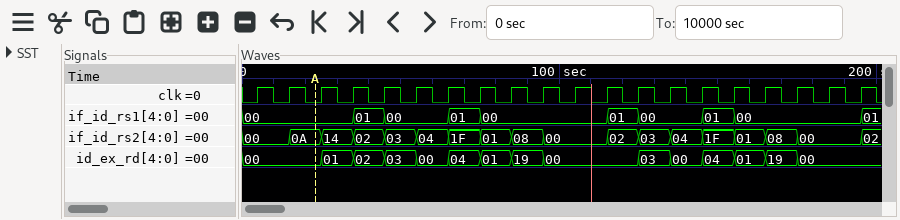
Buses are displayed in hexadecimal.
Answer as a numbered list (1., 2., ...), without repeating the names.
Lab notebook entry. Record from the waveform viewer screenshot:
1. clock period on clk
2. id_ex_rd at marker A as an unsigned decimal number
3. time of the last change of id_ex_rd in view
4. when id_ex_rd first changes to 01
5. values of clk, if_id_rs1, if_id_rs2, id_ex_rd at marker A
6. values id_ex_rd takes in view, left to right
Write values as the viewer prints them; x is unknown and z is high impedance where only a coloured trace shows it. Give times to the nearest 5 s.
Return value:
1. 10 s
2. 0
3. 175 s
4. 25 s
5. clk=0, if_id_rs1=00, if_id_rs2=0A, id_ex_rd=00
6. 00, 01, 02, 03, 00, 04, 01, 19, 00, 03, 00, 04, 01, 19, 00
